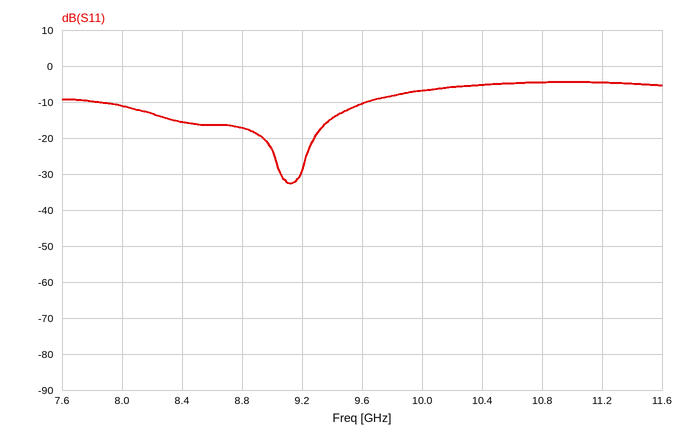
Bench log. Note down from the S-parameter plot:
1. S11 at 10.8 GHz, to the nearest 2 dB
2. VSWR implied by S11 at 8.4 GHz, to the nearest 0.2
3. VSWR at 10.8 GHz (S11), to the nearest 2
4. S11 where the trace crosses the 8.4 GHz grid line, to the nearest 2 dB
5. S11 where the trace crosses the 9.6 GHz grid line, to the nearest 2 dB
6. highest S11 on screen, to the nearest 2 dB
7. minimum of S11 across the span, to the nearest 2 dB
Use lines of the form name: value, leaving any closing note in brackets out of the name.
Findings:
S11 at 10.8 GHz, to the nearest 2 dB: -4 dB
VSWR implied by S11 at 8.4 GHz, to the nearest 0.2: 1.4
VSWR at 10.8 GHz (S11), to the nearest 2: 4
S11 where the trace crosses the 8.4 GHz grid line, to the nearest 2 dB: -16 dB
S11 where the trace crosses the 9.6 GHz grid line, to the nearest 2 dB: -10 dB
highest S11 on screen, to the nearest 2 dB: -4 dB
minimum of S11 across the span, to the nearest 2 dB: -32 dB
